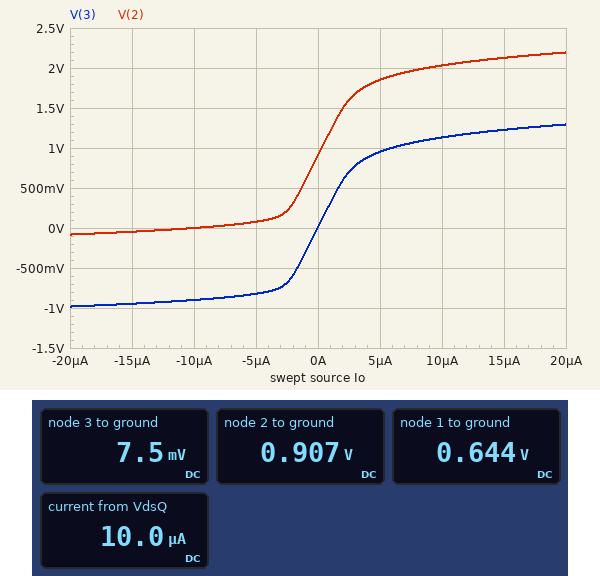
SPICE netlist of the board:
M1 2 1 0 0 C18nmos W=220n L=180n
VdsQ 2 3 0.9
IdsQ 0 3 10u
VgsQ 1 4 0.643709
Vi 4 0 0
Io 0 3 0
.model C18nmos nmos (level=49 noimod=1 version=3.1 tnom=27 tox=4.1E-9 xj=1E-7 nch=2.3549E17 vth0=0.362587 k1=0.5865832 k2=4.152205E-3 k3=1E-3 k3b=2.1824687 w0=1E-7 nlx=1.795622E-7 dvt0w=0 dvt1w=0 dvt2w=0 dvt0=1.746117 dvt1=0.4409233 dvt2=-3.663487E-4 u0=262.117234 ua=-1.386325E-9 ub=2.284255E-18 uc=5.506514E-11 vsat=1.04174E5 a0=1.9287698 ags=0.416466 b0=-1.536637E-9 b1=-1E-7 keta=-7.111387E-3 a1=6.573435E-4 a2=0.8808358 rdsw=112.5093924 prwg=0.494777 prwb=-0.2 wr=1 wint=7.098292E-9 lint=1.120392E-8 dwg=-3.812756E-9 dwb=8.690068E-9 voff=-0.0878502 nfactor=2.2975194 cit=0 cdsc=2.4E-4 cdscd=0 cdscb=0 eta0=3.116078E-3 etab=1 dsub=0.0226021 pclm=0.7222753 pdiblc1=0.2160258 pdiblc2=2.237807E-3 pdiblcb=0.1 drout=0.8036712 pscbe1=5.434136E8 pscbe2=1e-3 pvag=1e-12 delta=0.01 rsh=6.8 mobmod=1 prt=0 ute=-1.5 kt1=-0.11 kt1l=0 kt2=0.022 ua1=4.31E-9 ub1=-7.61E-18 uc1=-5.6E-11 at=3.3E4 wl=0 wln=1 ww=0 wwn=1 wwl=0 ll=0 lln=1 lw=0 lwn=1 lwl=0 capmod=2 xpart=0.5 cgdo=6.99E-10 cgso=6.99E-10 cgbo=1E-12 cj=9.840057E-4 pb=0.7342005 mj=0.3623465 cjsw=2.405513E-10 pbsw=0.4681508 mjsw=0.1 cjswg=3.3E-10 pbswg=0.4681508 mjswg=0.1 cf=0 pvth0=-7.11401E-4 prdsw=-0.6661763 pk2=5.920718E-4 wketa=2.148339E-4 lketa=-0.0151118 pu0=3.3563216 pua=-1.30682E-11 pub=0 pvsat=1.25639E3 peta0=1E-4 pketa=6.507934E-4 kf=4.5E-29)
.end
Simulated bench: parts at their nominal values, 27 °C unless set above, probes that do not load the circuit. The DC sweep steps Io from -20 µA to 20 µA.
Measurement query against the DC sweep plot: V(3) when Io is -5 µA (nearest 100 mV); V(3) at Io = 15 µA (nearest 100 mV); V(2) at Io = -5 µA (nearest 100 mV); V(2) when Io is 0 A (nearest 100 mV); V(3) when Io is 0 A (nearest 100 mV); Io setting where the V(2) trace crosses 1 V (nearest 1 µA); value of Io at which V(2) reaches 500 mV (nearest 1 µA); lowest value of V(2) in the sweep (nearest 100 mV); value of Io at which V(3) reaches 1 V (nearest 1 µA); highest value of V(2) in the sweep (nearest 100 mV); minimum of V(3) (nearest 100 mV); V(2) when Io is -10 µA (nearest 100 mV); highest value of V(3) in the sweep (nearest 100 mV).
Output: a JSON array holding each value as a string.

["-800 mV", "1.2 V", "100 mV", "900 mV", "0 V", "0 A", "-1 µA", "-100 mV", "6 µA", "2.2 V", "-1.0 V", "0 V", "1.3 V"]
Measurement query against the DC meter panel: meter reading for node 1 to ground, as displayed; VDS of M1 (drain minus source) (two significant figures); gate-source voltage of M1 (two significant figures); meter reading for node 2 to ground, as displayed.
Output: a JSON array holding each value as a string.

["0.644 V", "910 mV", "640 mV", "0.907 V"]
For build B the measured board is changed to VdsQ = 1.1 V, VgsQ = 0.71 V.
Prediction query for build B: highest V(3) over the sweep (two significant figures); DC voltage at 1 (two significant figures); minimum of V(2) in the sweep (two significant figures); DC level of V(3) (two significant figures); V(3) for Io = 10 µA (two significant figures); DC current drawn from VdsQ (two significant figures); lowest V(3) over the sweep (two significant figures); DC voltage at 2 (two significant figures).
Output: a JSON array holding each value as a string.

["950 mV", "710 mV", "-67 mV", "-980 mV", "550 mV", "10 µA", "-1.2 V", "120 mV"]
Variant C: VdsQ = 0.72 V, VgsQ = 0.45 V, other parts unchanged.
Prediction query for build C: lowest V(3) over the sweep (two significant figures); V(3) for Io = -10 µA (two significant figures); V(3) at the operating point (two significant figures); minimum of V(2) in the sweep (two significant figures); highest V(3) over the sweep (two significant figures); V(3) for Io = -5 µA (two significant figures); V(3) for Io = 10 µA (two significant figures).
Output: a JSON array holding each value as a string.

["-870 mV", "-720 mV", "1.8 V", "-150 mV", "2.1 V", "1.6 V", "2.0 V"]
